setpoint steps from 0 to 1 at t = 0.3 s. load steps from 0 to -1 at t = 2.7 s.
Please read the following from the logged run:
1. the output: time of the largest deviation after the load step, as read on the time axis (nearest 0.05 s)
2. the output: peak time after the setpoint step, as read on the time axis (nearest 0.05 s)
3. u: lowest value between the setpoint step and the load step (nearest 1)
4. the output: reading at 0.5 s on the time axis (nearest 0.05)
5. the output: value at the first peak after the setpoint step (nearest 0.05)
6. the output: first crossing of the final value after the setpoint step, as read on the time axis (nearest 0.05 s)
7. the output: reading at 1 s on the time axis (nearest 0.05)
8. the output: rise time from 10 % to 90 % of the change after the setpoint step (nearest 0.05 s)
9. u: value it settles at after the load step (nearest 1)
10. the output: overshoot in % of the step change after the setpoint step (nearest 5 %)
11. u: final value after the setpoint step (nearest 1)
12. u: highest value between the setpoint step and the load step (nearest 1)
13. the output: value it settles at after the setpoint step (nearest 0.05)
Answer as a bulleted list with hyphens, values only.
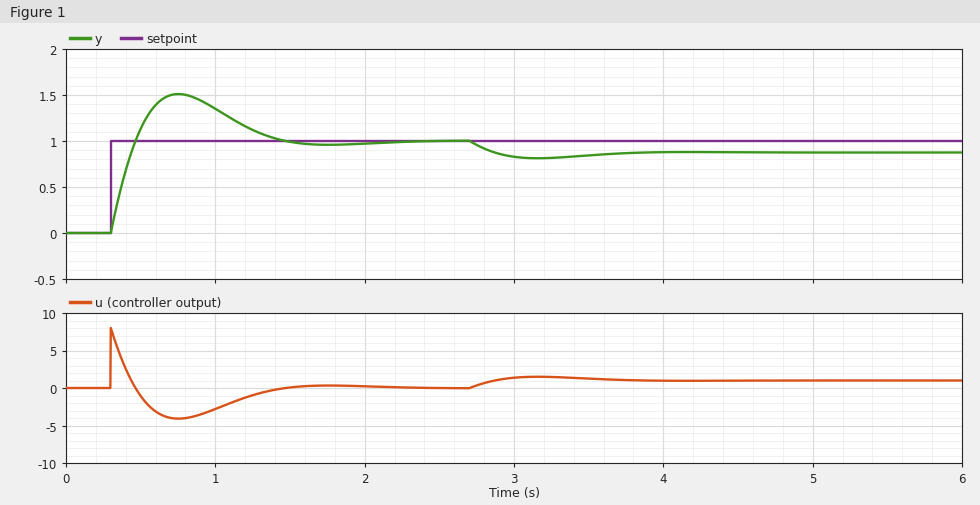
- 3.15 s
- 0.75 s
- -4
- 1.15
- 1.50
- 0.45 s
- 1.35
- 0.15 s
- 1
- 50 %
- 0
- 8
- 1.00
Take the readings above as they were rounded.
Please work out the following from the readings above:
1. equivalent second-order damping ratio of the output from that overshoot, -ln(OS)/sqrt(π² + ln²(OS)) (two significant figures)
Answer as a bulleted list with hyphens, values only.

- 0.22
